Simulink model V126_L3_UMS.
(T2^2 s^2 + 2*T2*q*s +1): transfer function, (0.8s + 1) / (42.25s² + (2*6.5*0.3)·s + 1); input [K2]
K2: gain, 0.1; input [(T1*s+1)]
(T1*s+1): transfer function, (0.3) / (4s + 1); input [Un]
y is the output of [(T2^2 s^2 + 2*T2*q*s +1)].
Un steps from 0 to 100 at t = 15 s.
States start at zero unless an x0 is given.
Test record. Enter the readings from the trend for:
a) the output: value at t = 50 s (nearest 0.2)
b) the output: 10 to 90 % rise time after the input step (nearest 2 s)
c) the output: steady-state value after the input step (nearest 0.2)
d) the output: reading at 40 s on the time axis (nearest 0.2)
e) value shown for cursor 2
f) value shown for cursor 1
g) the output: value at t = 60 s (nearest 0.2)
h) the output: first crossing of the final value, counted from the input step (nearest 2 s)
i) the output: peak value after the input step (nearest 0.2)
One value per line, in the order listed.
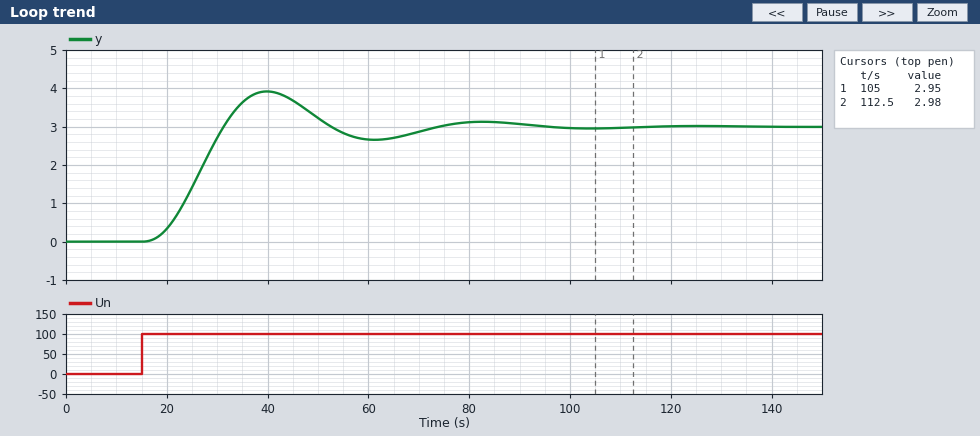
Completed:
3.2
10 s
3.0
4.0
2.98
2.95
2.6
16 s
4.0
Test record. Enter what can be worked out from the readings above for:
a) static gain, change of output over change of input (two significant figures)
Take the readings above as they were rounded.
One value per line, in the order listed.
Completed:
0.030
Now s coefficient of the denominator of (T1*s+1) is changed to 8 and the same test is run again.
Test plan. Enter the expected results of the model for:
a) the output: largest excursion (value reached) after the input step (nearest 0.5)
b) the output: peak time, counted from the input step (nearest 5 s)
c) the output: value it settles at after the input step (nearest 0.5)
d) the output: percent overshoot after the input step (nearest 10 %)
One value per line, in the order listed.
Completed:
3.5
30 s
3.0
20 %
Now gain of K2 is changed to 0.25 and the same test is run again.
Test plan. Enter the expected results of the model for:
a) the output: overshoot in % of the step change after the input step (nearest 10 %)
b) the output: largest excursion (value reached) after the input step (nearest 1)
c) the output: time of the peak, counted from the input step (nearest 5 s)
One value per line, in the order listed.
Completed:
30 %
10
25 s
